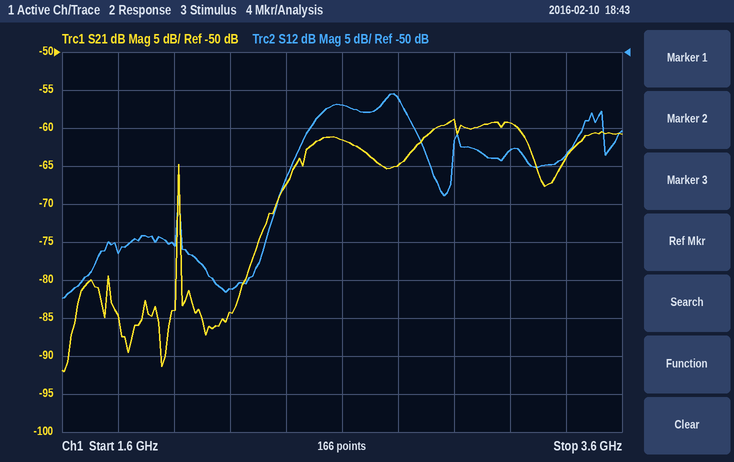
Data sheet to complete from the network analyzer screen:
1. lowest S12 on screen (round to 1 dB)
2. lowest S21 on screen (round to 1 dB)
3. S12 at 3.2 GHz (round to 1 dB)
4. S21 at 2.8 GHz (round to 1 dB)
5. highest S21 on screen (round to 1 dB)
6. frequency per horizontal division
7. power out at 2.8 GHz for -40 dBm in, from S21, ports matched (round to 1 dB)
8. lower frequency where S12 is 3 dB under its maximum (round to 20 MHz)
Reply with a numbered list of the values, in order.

1. -82 dB
2. -92 dB
3. -63 dB
4. -65 dB
5. -59 dB
6. 200 MHz
7. -105 dBm
8. 2.52 GHz
